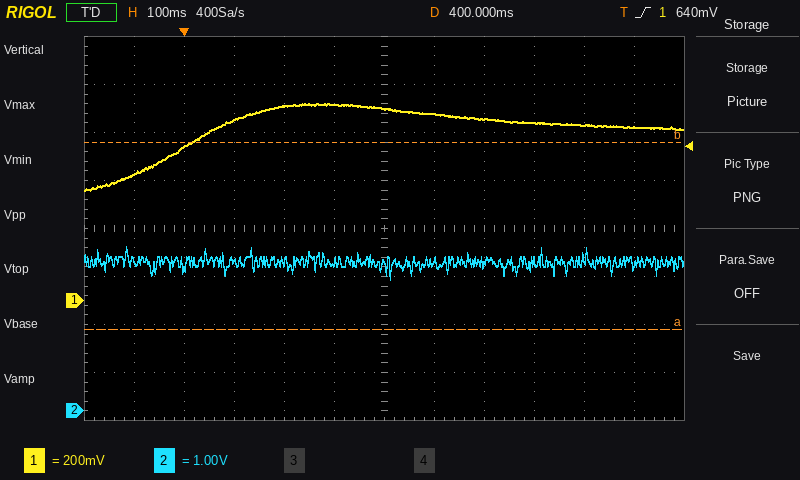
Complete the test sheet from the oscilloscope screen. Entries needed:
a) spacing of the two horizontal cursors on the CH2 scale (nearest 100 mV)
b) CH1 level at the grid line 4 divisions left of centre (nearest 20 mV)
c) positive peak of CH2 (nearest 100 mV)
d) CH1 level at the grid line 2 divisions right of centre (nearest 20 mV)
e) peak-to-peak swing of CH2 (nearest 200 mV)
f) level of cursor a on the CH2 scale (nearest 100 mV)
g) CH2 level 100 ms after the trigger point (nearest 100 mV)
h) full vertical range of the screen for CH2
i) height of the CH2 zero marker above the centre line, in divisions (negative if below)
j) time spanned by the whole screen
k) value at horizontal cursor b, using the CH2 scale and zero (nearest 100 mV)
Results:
3.9 V
640 mV
3.4 V
760 mV
600 mV
1.7 V
3.1 V
8 V
-3.8 div
1.2 s
5.6 V
